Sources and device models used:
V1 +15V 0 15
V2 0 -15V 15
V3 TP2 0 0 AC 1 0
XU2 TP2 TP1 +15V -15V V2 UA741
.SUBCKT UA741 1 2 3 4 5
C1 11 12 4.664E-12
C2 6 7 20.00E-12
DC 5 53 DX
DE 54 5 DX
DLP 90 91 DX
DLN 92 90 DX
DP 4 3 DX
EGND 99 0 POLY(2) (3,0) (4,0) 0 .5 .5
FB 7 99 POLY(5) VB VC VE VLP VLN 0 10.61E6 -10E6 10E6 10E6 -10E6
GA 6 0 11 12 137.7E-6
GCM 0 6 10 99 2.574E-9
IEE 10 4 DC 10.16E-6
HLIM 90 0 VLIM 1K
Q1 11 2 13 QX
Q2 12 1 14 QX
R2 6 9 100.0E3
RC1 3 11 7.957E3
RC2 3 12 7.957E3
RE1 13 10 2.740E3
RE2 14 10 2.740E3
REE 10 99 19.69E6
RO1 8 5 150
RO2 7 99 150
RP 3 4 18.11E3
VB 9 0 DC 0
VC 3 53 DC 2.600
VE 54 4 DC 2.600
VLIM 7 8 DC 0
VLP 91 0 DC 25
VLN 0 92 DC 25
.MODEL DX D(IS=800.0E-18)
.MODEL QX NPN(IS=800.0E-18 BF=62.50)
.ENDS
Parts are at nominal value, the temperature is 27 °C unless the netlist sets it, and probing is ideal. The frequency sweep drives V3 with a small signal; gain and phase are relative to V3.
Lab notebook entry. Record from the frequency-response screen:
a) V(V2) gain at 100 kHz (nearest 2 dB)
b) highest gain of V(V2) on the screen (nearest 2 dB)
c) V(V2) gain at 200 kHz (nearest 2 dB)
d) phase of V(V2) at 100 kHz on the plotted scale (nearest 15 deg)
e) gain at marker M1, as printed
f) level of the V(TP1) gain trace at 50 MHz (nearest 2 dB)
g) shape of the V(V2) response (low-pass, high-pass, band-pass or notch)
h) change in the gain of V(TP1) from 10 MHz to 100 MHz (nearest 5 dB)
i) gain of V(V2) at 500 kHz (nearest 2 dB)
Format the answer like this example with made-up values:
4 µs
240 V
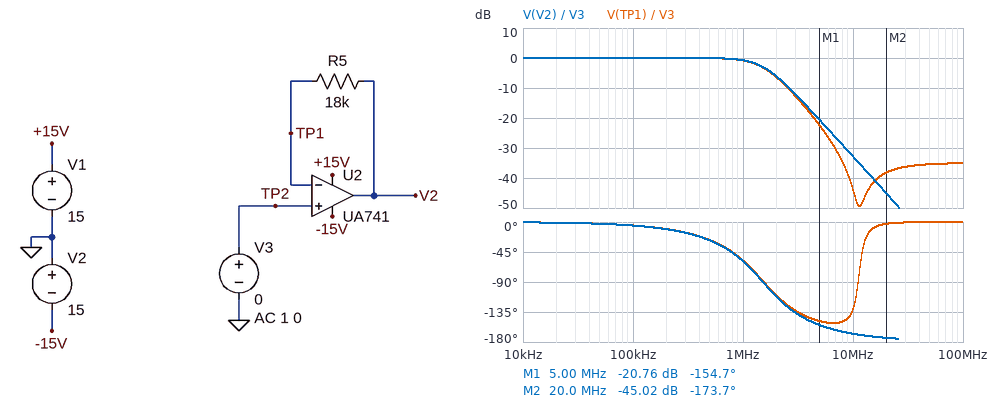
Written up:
0 dB
0 dB
0 dB
0 deg
-20.76 dB
-36 dB
low-pass
10 dB
0 dB
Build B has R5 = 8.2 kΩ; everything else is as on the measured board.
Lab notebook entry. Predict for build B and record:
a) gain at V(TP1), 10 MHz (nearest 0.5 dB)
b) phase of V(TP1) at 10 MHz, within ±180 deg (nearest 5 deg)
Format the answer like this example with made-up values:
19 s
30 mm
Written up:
-36.5 dB
-160 deg
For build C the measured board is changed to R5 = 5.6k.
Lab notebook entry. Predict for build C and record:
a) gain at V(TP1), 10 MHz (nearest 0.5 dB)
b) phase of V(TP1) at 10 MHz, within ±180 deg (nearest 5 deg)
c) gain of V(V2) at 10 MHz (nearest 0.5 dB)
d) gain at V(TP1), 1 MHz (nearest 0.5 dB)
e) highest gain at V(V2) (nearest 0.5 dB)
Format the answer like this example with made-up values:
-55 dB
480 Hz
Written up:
-35.0 dB
-165 deg
-32.5 dB
-0.5 dB
0 dB
